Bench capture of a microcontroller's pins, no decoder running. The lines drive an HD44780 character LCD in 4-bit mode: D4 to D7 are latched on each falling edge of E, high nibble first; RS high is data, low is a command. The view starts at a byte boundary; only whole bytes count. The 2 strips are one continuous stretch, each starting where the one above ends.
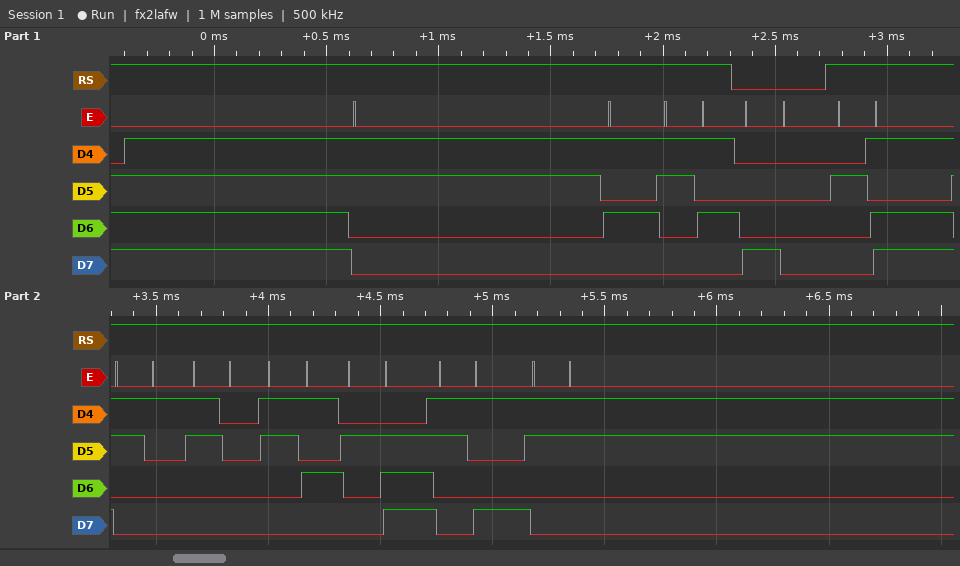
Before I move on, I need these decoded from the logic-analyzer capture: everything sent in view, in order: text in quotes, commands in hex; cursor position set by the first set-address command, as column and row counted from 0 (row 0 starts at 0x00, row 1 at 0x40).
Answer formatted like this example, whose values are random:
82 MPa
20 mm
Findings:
"55" 0x80 "-105.93"
column 0, row 0
